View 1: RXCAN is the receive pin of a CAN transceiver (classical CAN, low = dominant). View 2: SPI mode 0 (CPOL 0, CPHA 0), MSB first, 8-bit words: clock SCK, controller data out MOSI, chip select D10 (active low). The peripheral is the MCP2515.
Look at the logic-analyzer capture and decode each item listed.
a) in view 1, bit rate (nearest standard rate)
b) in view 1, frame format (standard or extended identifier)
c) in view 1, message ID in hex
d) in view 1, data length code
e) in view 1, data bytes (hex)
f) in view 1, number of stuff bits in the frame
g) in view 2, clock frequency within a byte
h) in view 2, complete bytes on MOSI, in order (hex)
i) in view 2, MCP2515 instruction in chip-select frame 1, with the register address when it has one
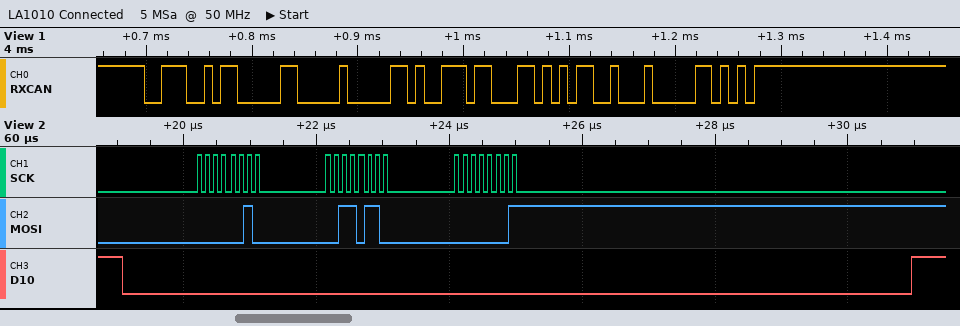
125 kbit/s
standard
0x396
4
00 A7 63 56
4
8 MHz
02 36 01
WRITE 0x36
